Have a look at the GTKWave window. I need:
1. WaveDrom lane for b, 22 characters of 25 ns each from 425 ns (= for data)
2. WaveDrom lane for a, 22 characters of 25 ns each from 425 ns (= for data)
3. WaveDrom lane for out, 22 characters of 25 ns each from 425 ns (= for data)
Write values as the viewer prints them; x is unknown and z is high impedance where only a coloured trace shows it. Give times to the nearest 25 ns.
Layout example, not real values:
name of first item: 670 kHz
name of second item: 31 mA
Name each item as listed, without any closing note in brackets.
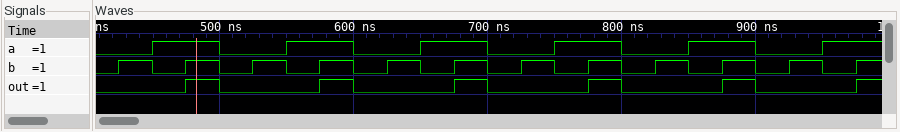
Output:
WaveDrom lane for b, 22 characters of 25 ns each from 425 ns: {name: 'b', wave: '1010101010101010101010'}
WaveDrom lane for a, 22 characters of 25 ns each from 425 ns: {name: 'a', wave: '01.0.1.0.1.0.1.0.1.0.1'}
WaveDrom lane for out, 22 characters of 25 ns each from 425 ns: {name: 'out', wave: '0.10..10..10..10..10..'}
